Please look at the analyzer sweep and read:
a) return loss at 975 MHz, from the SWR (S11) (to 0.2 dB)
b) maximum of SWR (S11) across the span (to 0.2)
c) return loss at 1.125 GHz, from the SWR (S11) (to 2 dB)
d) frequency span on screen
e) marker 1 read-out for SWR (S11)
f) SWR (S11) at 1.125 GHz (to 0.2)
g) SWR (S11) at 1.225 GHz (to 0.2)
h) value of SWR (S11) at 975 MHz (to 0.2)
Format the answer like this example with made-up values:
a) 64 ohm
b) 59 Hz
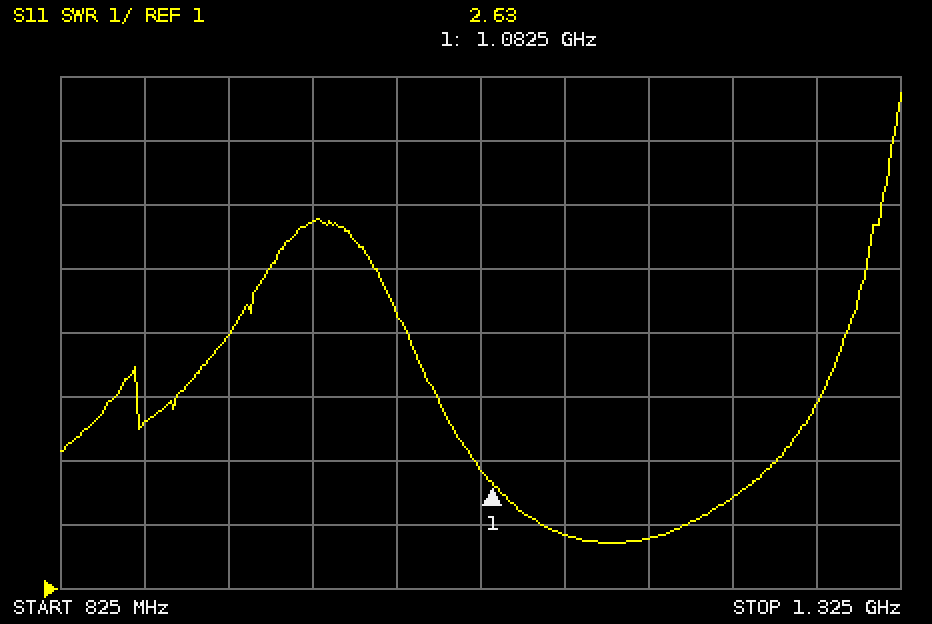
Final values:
a) 2.6 dB
b) 8.8
c) 10 dB
d) 500 MHz
e) 2.63
f) 1.8
g) 2.4
h) 6.8
